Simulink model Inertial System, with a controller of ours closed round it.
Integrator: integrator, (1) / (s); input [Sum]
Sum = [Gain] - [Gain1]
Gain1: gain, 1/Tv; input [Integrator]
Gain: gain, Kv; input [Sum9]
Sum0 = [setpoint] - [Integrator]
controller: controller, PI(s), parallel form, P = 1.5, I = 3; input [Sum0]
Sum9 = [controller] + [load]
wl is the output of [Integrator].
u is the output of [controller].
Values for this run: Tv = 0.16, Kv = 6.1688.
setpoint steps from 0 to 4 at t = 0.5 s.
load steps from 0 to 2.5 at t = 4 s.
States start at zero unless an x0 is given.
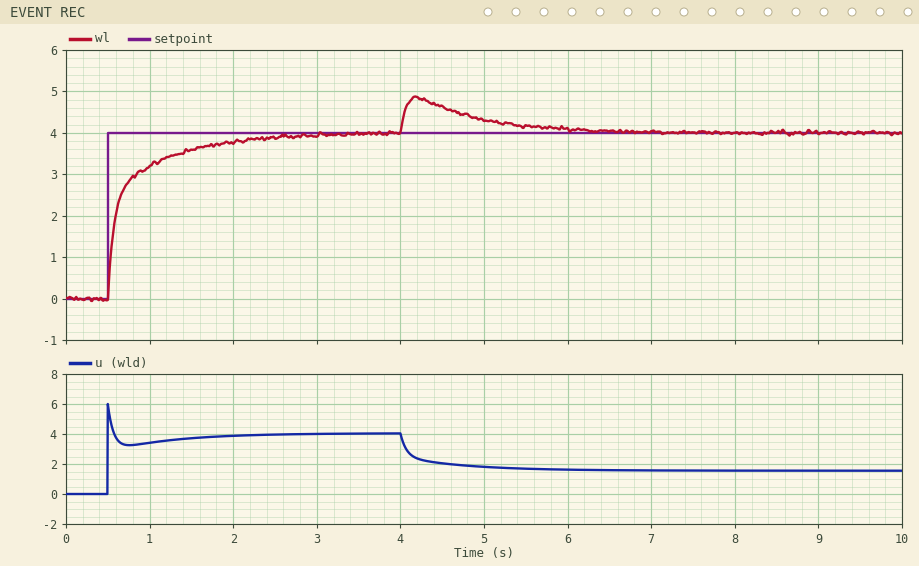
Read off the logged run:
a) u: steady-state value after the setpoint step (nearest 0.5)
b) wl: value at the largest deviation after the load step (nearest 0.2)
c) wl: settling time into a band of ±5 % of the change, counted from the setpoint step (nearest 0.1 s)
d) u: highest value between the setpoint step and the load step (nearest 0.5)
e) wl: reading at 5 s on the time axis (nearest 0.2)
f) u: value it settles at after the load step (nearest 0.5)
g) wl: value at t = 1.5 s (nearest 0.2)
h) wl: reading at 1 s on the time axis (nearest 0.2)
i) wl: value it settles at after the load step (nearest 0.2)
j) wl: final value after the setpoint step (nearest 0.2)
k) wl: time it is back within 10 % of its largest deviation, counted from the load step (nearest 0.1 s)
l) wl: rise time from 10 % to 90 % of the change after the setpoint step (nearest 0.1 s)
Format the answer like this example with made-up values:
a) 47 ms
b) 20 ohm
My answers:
a) 4.0
b) 4.8
c) 1.6 s
d) 6.0
e) 4.4
f) 1.5
g) 3.6
h) 3.2
i) 4.0
j) 4.0
k) 2.0 s
l) 1.0 s
